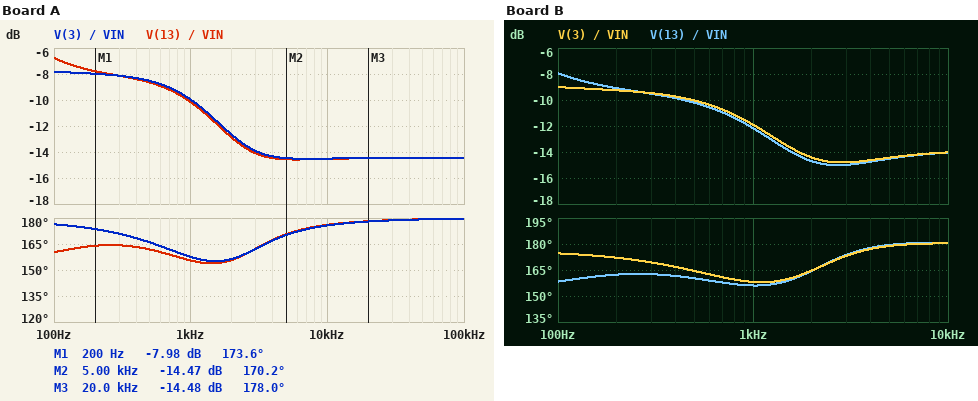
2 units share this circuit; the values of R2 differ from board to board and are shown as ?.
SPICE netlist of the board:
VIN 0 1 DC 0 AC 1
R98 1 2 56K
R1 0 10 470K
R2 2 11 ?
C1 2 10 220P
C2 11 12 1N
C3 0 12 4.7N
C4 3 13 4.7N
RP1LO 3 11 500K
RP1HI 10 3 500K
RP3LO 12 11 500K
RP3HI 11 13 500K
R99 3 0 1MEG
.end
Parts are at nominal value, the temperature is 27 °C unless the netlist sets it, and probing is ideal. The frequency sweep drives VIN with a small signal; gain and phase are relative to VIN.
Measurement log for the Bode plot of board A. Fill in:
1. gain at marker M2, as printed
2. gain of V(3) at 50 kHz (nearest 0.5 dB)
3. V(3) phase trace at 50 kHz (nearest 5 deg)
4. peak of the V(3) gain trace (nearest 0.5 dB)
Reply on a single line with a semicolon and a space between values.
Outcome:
-14.47 dB; -14.5 dB; 180 deg; -8.0 dB
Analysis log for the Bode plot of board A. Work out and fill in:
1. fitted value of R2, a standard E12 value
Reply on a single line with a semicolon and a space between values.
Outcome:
180 kΩ
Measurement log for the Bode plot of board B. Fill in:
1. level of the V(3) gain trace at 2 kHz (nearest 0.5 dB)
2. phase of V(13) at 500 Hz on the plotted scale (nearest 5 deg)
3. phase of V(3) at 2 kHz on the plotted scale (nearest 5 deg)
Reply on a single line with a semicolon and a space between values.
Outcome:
-14.5 dB; 160 deg; 165 deg
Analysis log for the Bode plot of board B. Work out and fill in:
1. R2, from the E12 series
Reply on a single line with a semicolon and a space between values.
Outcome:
270 kΩ
